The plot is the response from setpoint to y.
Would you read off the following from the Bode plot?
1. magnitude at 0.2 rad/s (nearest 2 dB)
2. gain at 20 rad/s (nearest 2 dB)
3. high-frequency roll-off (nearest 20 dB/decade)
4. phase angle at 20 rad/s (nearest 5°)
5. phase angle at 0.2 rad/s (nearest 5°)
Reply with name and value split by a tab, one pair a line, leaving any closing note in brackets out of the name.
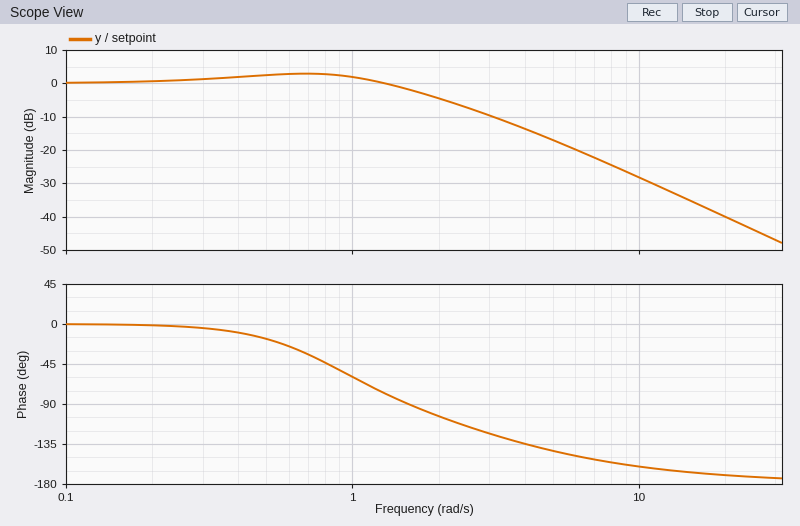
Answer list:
magnitude at 0.2 rad/s	0 dB
gain at 20 rad/s	-40 dB
high-frequency roll-off	-40 dB/decade
phase angle at 20 rad/s	-170°
phase angle at 0.2 rad/s	0°
